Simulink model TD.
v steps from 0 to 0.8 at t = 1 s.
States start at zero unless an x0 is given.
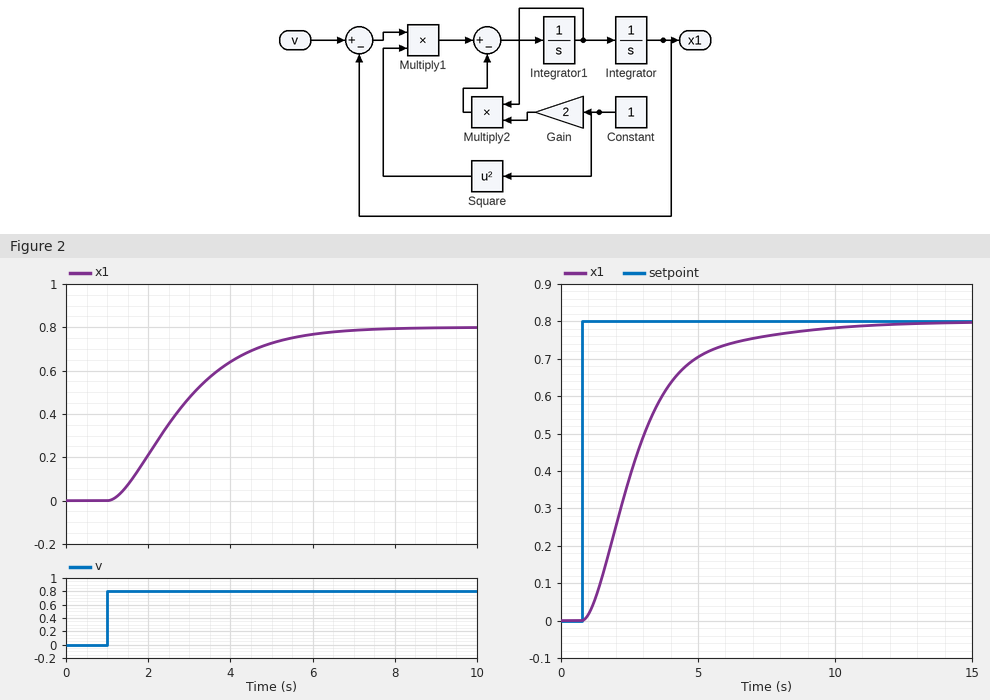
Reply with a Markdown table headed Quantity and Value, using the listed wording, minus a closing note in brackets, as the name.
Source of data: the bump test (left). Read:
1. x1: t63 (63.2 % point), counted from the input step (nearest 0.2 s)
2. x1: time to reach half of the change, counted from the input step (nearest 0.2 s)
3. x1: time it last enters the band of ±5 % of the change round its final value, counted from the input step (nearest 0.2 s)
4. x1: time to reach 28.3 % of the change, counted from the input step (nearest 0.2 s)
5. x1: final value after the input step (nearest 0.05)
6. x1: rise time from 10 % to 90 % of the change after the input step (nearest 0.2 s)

| Quantity | Value |
|---|---|
| x1: t63 (63.2 % point), counted from the input step | 2.2 s |
| x1: time to reach half of the change, counted from the input step | 1.6 s |
| x1: time it last enters the band of ±5 % of the change round its final value, counted from the input step | 4.8 s |
| x1: time to reach 28.3 % of the change, counted from the input step | 1.0 s |
| x1: final value after the input step | 0.80 |
| x1: rise time from 10 % to 90 % of the change after the input step | 3.4 s |
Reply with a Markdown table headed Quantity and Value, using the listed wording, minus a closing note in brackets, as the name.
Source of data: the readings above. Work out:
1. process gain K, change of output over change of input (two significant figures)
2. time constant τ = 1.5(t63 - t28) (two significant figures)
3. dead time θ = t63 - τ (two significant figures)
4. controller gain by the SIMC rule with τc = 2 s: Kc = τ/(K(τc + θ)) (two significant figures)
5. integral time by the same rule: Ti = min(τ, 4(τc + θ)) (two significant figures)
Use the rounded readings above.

| Quantity | Value |
|---|---|
| process gain K, change of output over change of input | 1.0 |
| time constant τ = 1.5(t63 - t28) | 1.8 s |
| dead time θ = t63 - τ | 0.40 s |
| controller gain by the SIMC rule with τc = 2 s: Kc = τ/(K(τc + θ)) | 0.75 |
| integral time by the same rule: Ti = min(τ, 4(τc + θ)) | 1.8 s |
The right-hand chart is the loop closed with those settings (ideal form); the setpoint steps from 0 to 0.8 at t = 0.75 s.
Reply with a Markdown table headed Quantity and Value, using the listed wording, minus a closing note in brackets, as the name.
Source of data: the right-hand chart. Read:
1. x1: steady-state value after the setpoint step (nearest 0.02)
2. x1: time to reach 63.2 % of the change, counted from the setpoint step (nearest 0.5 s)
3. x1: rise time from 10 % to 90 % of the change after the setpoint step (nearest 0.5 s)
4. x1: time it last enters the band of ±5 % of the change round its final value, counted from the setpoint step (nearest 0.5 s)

| Quantity | Value |
|---|---|
| x1: steady-state value after the setpoint step | 0.80 |
| x1: time to reach 63.2 % of the change, counted from the setpoint step | 2.5 s |
| x1: rise time from 10 % to 90 % of the change after the setpoint step | 4.0 s |
| x1: time it last enters the band of ±5 % of the change round its final value, counted from the setpoint step | 6.5 s |
